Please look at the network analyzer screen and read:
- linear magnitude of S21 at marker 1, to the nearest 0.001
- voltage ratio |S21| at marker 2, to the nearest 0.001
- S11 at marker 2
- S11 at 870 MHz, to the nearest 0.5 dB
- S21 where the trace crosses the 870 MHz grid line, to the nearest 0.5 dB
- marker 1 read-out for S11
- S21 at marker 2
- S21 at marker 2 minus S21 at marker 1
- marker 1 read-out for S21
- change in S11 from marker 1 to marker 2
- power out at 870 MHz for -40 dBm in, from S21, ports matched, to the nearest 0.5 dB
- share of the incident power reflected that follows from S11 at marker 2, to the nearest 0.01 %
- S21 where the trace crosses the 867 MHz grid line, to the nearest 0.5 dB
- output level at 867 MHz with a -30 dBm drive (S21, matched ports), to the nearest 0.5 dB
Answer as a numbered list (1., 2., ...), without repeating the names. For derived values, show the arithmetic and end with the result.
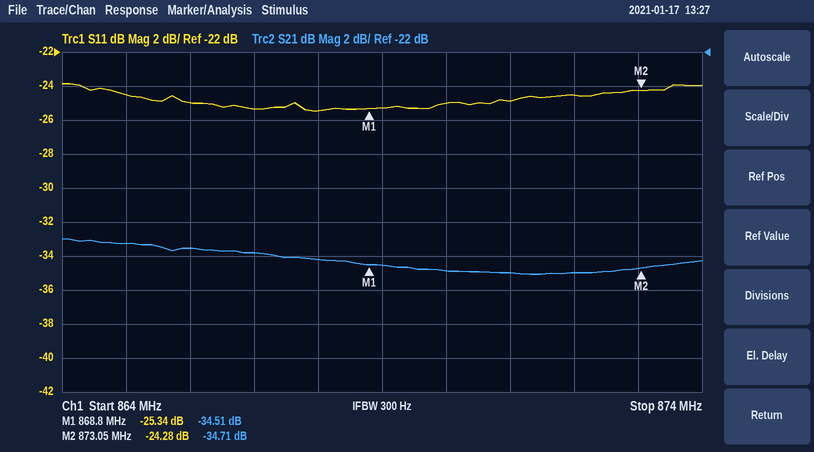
1. 10^(-34.51/20) ≈ 0.019
2. 10^(-34.71/20) ≈ 0.018
3. -24.28 dB
4. -25.0 dB
5. -35.0 dB
6. -25.34 dB
7. -34.71 dB
8. -34.71 − (-34.51) = -0.20 dB
9. -34.51 dB
10. -24.28 − (-25.34) = 1.06 dB
11. -40 dBm + (-35.0 dB) = -75.0 dBm
12. 10^(-24.28/10) ≈ 0.37 %
13. -34.0 dB
14. -30 dBm + (-34.0 dB) = -64.0 dBm
